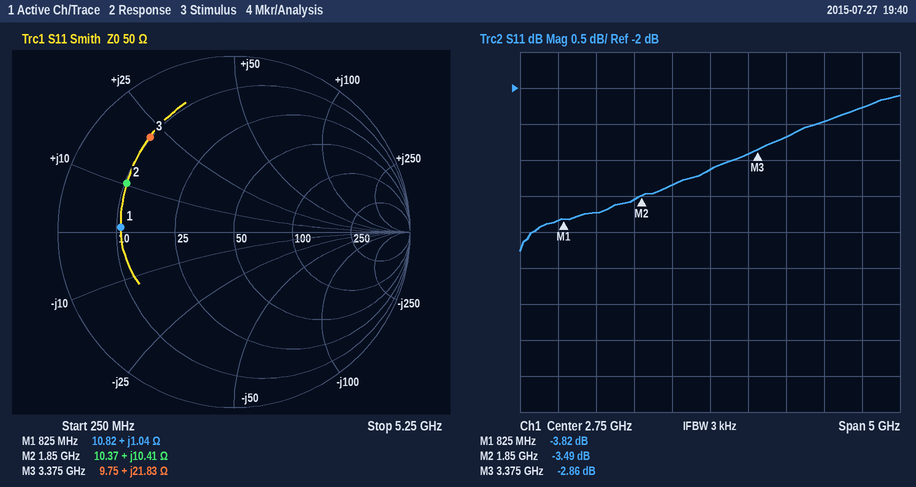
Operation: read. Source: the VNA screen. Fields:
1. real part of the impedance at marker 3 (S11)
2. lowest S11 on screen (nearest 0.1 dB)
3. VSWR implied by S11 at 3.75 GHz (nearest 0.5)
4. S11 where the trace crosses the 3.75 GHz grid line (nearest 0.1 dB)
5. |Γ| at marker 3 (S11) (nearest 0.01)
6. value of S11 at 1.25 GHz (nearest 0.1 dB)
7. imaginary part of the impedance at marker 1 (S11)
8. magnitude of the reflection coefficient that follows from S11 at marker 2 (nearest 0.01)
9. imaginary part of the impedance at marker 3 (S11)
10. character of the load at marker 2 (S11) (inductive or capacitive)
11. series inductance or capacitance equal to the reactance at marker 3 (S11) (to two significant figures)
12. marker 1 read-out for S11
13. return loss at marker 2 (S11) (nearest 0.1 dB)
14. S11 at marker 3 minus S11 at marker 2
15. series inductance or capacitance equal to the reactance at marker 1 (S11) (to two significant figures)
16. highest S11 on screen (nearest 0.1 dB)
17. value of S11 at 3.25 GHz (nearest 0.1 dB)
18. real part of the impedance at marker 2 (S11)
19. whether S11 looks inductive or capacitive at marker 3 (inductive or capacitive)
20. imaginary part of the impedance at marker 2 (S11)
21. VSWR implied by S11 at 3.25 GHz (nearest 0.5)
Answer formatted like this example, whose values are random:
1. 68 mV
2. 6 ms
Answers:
1. 9.75 Ω
2. -4.3 dB
3. 6.5
4. -2.7 dB
5. 0.72
6. -3.7 dB
7. +1.04 Ω
8. 0.67
9. +21.83 Ω
10. inductive
11. 1.0 nH
12. -3.82 dB
13. 3.5 dB
14. 0.63 dB
15. 200 pH
16. -2.1 dB
17. -2.9 dB
18. 10.37 Ω
19. inductive
20. +10.41 Ω
21. 6.0
